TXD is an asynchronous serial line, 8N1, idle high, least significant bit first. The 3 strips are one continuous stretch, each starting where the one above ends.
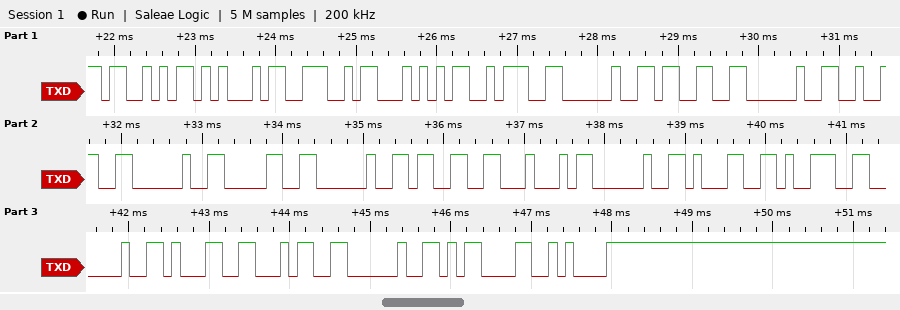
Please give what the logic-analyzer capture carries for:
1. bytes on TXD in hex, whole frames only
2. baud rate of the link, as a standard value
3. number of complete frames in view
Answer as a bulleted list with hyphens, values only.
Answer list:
- 53 45 4E 54 3A 20 33 20 32 20 30 20 33 44 20 31 39 20 31 34 20 0D 0A
- 9600 baud
- 23
